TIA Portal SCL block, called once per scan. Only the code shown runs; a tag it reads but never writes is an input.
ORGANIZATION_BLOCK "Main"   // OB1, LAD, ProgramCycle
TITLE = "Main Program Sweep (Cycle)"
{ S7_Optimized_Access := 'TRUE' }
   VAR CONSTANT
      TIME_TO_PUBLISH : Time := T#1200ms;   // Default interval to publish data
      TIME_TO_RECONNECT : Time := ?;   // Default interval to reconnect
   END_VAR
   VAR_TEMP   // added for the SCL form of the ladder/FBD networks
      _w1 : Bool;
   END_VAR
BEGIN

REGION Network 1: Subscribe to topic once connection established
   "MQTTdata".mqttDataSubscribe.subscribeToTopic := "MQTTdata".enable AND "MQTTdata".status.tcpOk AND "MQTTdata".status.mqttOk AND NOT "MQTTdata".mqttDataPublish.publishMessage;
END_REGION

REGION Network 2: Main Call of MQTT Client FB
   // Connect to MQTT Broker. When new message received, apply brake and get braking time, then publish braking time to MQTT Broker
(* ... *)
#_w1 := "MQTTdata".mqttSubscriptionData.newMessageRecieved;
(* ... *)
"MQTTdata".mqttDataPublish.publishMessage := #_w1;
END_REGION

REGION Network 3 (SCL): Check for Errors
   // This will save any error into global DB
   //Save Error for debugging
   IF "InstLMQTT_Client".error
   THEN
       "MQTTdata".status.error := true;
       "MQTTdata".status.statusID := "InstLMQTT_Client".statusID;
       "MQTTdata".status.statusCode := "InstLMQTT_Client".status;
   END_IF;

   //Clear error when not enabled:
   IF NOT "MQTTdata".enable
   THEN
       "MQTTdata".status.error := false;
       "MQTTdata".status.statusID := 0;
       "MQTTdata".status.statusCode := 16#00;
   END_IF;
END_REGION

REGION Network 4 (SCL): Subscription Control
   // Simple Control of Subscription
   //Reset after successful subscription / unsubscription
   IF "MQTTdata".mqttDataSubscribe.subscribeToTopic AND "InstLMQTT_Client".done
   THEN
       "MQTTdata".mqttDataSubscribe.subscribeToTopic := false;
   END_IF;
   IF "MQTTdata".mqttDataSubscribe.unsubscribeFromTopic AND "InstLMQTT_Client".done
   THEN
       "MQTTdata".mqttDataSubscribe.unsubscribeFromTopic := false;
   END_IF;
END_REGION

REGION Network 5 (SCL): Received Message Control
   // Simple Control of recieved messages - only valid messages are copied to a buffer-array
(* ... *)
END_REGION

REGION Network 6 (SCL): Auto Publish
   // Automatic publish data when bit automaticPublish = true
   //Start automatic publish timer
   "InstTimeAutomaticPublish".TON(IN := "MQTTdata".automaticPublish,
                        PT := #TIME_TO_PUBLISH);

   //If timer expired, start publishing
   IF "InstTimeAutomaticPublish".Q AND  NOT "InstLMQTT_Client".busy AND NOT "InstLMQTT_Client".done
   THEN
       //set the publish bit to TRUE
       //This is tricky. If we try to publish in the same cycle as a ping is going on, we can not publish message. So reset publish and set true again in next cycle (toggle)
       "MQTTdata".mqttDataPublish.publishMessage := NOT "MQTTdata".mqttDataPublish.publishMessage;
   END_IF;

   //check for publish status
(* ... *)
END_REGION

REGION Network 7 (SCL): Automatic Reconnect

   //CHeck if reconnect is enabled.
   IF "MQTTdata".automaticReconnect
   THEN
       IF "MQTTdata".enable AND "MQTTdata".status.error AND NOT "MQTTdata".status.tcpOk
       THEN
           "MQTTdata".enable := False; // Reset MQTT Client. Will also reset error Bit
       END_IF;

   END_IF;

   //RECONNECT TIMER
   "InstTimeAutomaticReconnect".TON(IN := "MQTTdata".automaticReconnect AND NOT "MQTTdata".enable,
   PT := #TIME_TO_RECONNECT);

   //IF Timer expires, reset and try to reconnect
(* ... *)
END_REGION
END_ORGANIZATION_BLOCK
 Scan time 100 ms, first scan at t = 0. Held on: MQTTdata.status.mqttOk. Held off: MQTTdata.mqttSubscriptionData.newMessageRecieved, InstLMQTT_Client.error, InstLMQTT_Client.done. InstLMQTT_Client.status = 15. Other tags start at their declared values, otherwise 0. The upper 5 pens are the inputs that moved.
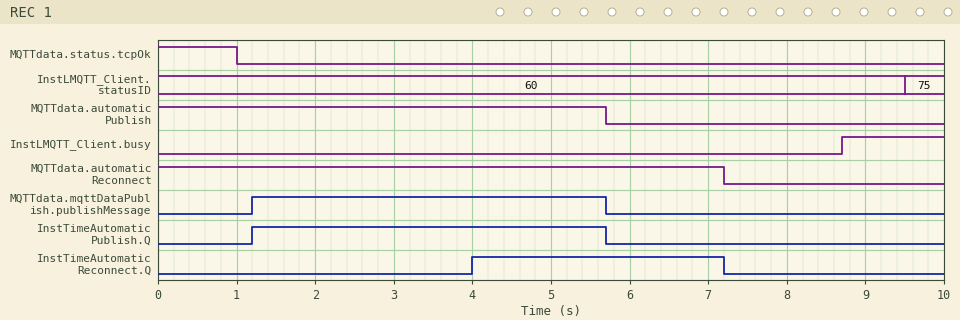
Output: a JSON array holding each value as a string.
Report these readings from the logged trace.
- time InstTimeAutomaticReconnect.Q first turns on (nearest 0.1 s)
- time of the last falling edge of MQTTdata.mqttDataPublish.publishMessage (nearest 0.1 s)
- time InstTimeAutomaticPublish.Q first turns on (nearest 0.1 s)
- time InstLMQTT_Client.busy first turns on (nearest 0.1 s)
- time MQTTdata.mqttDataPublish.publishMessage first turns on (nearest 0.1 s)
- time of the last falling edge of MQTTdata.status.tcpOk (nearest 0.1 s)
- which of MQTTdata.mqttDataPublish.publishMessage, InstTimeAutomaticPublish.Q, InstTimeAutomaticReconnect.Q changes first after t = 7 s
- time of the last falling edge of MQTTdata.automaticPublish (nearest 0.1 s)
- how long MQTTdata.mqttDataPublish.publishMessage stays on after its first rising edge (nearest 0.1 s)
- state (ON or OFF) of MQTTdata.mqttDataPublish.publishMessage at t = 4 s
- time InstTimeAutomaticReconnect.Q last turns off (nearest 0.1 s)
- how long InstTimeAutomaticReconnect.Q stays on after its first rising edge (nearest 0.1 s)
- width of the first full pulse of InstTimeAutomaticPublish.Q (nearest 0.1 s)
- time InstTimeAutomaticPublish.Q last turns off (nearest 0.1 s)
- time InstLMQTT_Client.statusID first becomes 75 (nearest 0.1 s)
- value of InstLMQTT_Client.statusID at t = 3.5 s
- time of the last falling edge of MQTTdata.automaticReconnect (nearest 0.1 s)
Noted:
["4.0 s", "5.7 s", "1.2 s", "8.7 s", "1.2 s", "1.0 s", "InstTimeAutomaticReconnect.Q", "5.7 s", "4.5 s", "ON", "7.2 s", "3.2 s", "4.5 s", "5.7 s", "9.5 s", "60", "7.2 s"]
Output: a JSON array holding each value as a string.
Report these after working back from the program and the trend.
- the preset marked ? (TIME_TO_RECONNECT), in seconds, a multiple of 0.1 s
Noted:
["4.0 s"]
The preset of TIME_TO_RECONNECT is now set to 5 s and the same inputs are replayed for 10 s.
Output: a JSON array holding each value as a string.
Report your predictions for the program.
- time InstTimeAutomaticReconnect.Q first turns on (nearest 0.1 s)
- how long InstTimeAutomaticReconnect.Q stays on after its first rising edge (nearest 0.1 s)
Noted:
["5.0 s", "2.2 s"]
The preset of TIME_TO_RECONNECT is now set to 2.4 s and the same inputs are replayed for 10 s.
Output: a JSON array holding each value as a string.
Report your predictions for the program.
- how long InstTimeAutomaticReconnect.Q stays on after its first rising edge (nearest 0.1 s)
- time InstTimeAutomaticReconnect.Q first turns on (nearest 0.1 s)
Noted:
["4.8 s", "2.4 s"]
